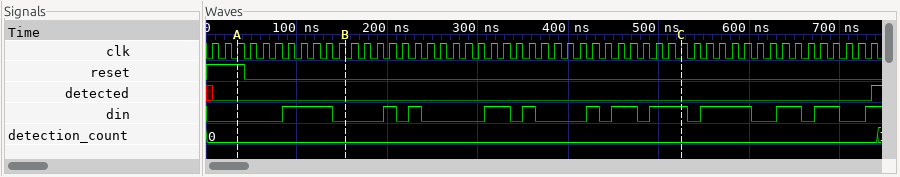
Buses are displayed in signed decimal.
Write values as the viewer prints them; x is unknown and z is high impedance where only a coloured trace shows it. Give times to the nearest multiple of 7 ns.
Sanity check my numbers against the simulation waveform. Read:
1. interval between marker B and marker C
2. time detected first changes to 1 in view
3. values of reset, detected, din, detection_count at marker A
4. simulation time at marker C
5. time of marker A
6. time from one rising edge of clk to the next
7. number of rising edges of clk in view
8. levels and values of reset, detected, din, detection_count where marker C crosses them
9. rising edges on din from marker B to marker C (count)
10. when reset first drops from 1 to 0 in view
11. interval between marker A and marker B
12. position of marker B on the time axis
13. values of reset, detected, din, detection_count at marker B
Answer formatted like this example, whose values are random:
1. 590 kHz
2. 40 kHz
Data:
1. 371 ns
2. 735 ns
3. reset=1, detected=0, din=0, detection_count=0
4. 525 ns
5. 35 ns
6. 14 ns
7. 53
8. reset=0, detected=0, din=1, detection_count=0
9. 7
10. 42 ns
11. 119 ns
12. 154 ns
13. reset=0, detected=0, din=0, detection_count=0
